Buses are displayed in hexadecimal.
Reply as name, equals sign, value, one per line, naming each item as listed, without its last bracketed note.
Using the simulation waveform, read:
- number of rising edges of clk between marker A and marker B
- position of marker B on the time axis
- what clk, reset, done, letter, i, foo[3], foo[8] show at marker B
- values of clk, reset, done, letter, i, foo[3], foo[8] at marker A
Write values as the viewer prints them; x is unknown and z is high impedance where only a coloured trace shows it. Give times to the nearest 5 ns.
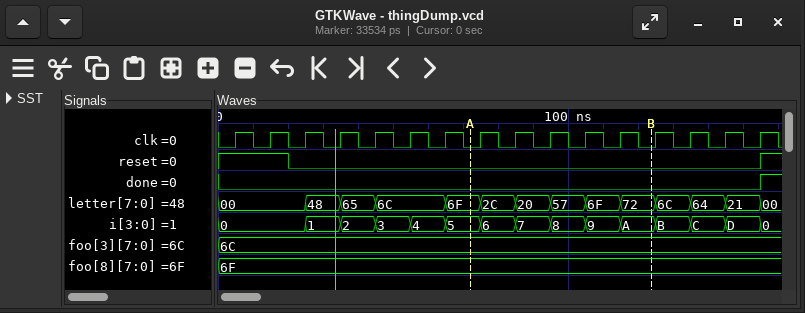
number of rising edges of clk between marker A and marker B = 5
position of marker B on the time axis = 125 ns
what clk, reset, done, letter, i, foo[3], foo[8] show at marker B = clk=0, reset=0, done=0, letter=72, i=A, foo[3]=6C, foo[8]=6F
values of clk, reset, done, letter, i, foo[3], foo[8] at marker A = clk=0, reset=0, done=0, letter=6F, i=5, foo[3]=6C, foo[8]=6F
